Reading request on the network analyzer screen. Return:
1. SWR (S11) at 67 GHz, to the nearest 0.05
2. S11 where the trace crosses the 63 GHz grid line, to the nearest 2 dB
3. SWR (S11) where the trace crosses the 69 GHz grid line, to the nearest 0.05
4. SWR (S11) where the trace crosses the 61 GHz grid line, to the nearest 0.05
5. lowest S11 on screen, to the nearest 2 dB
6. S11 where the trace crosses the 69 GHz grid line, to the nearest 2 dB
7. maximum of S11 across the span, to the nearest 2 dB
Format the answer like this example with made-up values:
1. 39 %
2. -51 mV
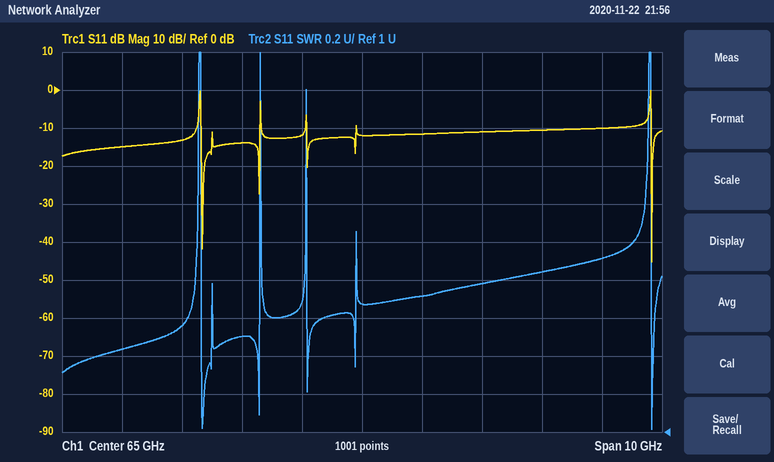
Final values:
1. 1.80
2. -14 dB
3. 1.90
4. 1.45
5. -46 dB
6. -10 dB
7. 0 dB
